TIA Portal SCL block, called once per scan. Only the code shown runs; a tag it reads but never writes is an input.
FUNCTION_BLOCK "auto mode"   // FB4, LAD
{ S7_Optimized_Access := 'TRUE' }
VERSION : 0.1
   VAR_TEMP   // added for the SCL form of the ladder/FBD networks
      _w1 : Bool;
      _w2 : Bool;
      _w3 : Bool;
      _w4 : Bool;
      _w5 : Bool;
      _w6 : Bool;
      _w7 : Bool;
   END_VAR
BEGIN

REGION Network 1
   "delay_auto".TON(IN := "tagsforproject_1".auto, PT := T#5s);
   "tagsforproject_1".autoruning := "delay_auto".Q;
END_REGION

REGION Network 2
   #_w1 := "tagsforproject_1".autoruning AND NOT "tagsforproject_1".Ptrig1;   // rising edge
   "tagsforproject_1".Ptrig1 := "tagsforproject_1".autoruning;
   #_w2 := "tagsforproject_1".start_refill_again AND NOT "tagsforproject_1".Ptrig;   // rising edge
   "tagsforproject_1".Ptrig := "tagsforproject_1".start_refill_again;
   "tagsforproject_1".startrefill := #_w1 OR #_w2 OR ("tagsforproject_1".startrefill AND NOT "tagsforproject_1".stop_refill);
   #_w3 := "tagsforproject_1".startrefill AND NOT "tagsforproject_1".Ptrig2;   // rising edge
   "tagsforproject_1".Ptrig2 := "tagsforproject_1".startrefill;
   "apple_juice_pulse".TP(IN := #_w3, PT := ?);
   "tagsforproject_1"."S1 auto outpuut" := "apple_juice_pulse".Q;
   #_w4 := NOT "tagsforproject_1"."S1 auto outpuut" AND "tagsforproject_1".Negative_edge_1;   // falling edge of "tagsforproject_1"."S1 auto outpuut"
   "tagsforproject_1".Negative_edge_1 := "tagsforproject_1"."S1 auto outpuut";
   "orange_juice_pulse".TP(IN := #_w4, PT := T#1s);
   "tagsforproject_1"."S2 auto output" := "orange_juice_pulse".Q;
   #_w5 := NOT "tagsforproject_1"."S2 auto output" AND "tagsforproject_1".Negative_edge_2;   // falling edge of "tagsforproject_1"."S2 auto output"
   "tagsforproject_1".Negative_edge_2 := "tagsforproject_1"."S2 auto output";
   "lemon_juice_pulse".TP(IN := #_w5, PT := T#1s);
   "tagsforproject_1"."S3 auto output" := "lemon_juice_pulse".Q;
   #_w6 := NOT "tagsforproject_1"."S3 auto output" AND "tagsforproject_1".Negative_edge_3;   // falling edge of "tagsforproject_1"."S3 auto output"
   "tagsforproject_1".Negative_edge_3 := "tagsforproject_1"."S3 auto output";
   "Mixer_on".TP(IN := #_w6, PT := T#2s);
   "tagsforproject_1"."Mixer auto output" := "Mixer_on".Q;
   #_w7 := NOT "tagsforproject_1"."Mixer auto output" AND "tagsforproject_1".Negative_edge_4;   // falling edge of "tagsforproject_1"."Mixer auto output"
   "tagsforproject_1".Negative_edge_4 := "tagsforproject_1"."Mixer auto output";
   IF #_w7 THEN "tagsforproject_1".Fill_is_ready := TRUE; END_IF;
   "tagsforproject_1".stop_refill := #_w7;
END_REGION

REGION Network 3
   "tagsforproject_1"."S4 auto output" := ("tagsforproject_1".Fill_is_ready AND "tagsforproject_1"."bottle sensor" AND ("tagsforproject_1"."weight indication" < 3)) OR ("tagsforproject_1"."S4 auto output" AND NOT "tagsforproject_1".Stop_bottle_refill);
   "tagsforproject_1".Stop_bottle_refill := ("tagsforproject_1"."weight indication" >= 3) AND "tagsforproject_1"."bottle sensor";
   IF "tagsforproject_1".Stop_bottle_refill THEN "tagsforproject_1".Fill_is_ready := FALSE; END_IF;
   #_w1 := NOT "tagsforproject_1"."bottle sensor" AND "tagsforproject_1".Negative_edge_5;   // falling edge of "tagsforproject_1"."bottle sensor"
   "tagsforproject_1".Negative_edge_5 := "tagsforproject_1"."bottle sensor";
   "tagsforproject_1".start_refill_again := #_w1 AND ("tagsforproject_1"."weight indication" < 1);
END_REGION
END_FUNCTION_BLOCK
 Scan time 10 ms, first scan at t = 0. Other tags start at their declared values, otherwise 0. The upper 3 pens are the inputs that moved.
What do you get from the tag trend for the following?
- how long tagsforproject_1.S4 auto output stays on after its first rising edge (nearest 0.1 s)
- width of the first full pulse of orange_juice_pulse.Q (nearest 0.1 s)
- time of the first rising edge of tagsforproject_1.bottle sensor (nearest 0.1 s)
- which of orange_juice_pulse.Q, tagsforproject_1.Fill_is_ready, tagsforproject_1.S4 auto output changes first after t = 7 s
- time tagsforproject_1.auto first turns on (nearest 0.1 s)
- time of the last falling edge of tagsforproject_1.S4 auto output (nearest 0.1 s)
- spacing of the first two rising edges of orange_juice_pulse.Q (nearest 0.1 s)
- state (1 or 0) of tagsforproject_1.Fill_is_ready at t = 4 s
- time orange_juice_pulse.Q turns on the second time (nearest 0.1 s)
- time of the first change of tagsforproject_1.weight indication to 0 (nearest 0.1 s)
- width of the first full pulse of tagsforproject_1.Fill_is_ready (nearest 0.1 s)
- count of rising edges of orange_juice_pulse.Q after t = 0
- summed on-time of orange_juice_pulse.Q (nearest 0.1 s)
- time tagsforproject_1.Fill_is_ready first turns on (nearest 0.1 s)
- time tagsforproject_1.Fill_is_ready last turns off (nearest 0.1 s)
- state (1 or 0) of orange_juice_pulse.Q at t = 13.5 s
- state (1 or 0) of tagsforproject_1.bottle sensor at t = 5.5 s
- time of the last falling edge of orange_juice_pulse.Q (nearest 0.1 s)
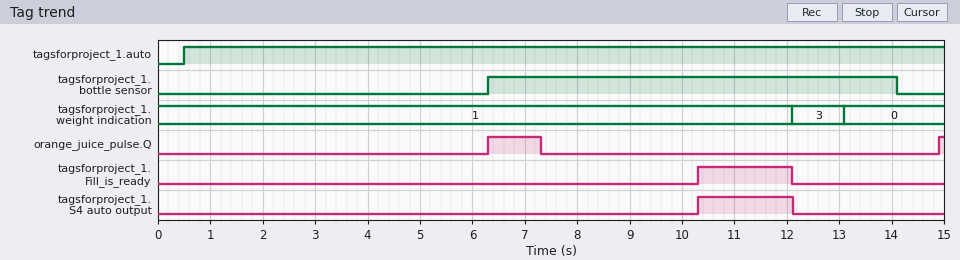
1.8 s
1.0 s
6.3 s
orange_juice_pulse.Q
0.5 s
12.1 s
8.6 s
0
14.9 s
13.1 s
1.8 s
2
1.1 s
10.3 s
12.1 s
0
0
7.3 s
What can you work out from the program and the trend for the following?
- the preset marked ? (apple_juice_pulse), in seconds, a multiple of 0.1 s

0.8 s
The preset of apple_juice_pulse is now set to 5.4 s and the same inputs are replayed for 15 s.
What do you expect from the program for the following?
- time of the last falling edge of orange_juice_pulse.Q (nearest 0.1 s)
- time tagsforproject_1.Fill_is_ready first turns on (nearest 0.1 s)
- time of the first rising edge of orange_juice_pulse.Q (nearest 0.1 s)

11.9 s
14.9 s
10.9 s
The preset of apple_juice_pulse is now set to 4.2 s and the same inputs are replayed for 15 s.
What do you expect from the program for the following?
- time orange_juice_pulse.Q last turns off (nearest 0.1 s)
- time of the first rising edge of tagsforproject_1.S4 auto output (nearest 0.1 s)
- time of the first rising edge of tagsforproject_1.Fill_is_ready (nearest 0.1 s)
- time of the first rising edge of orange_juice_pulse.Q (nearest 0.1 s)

10.7 s
13.7 s
13.7 s
9.7 s
